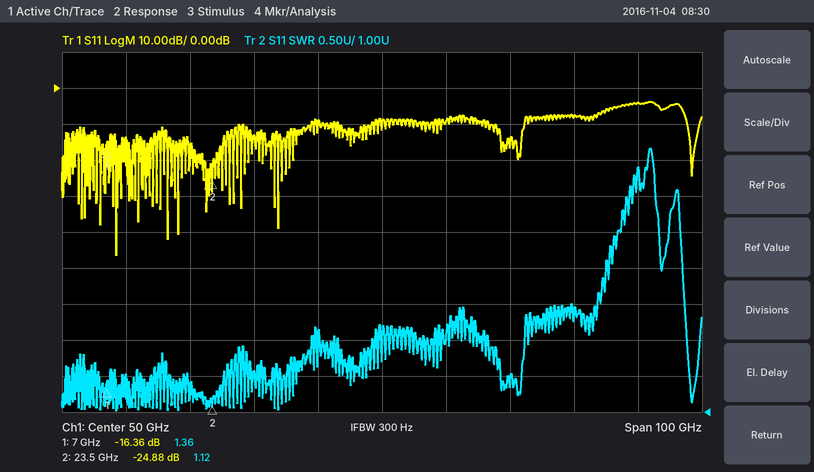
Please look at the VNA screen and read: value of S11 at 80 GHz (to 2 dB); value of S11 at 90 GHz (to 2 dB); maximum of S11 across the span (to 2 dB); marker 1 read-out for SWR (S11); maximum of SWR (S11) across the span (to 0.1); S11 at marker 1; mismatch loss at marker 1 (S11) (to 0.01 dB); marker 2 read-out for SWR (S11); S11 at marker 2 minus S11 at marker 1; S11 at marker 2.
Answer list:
-8 dB
-4 dB
-4 dB
1.36
4.7
-16.36 dB
0.10 dB
1.12
-8.52 dB
-24.88 dB
